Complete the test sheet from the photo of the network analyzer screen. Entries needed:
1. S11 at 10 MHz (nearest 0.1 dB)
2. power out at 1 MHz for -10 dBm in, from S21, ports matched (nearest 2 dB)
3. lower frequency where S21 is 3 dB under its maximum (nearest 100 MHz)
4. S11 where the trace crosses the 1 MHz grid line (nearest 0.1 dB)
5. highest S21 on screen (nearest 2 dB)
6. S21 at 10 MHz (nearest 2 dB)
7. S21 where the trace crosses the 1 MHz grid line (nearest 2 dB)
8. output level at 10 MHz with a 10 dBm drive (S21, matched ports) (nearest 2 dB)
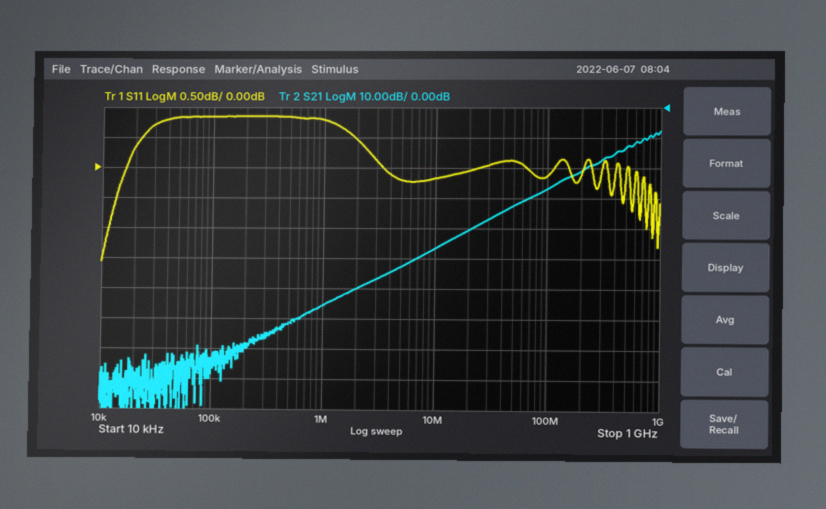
-0.2 dB
-76 dBm
700 MHz
0.8 dB
-8 dB
-46 dB
-66 dB
-36 dBm
